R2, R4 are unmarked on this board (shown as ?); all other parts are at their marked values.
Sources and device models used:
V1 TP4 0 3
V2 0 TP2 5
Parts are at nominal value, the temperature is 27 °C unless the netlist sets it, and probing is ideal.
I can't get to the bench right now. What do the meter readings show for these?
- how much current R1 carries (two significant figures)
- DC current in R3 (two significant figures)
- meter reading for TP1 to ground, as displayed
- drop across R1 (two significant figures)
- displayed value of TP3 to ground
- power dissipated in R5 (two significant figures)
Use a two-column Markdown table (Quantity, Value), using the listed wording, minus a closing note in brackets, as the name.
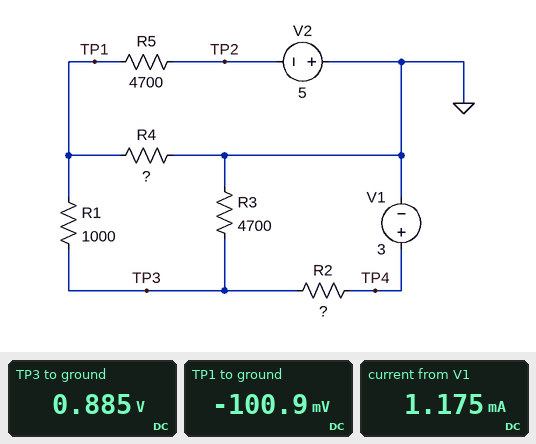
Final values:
| Quantity | Value |
|---|---|
| how much current R1 carries | 990 µA |
| DC current in R3 | 190 µA |
| meter reading for TP1 to ground, as displayed | -100.9 mV |
| drop across R1 | 990 mV |
| displayed value of TP3 to ground | 0.885 V |
| power dissipated in R5 | 5.1 mW |
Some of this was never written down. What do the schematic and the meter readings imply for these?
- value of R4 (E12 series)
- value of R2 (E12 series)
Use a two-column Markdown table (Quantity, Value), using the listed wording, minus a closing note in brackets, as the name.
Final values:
| Quantity | Value |
|---|---|
| value of R4 | 1.8 kΩ |
| value of R2 | 1.8 kΩ |
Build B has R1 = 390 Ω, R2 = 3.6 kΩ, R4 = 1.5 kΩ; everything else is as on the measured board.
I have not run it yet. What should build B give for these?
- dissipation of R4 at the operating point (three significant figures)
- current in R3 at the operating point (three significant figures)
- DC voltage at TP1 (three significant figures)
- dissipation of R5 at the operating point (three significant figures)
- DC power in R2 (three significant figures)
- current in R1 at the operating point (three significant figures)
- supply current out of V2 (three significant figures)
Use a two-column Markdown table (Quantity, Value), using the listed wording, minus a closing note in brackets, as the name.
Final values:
| Quantity | Value |
|---|---|
| dissipation of R4 at the operating point | 53.1 µW |
| current in R3 at the operating point | 7.65 µA |
| DC voltage at TP1 | -282 mV |
| dissipation of R5 at the operating point | 4.74 mW |
| DC power in R2 | 2.44 mW |
| current in R1 at the operating point | 816 µA |
| supply current out of V2 | 1.00 mA |
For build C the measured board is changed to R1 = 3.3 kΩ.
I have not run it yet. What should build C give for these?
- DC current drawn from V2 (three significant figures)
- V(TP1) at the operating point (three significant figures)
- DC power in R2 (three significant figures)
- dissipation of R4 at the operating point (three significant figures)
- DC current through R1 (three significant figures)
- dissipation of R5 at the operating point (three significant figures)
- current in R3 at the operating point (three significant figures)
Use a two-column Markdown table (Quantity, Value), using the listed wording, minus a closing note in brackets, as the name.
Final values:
| Quantity | Value |
|---|---|
| DC current drawn from V2 | 936 µA |
| V(TP1) at the operating point | -601 mV |
| DC power in R2 | 1.45 mW |
| dissipation of R4 at the operating point | 201 µW |
| DC current through R1 | 602 µA |
| dissipation of R5 at the operating point | 4.12 mW |
| current in R3 at the operating point | 295 µA |
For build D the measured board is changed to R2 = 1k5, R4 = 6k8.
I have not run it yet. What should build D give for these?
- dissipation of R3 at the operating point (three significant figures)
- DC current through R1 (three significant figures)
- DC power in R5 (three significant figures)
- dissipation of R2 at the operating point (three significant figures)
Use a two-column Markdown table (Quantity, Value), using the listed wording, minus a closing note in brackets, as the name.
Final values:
| Quantity | Value |
|---|---|
| dissipation of R3 at the operating point | 241 µW |
| DC current through R1 | 1.06 mA |
| DC power in R5 | 5.32 mW |
| dissipation of R2 at the operating point | 2.50 mW |
